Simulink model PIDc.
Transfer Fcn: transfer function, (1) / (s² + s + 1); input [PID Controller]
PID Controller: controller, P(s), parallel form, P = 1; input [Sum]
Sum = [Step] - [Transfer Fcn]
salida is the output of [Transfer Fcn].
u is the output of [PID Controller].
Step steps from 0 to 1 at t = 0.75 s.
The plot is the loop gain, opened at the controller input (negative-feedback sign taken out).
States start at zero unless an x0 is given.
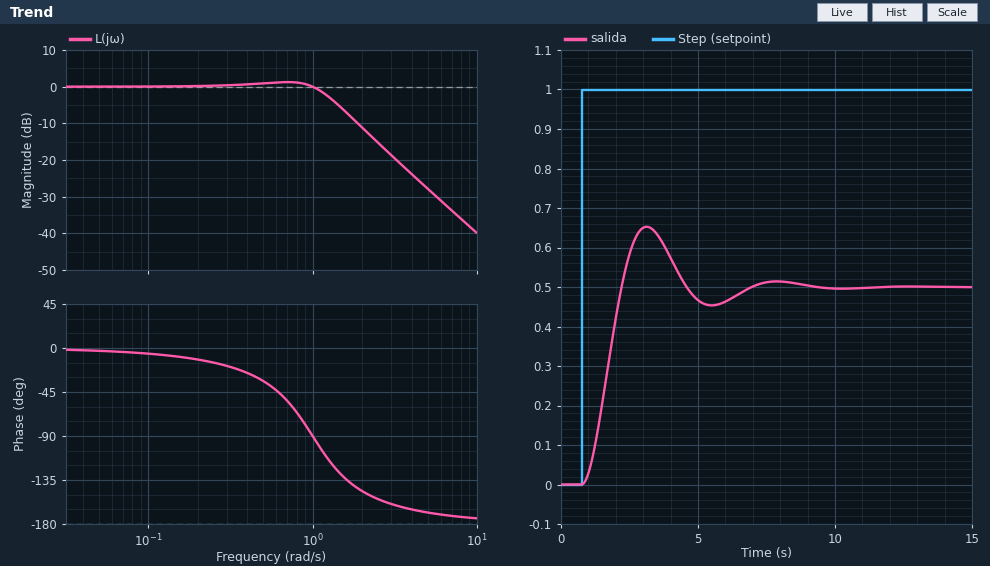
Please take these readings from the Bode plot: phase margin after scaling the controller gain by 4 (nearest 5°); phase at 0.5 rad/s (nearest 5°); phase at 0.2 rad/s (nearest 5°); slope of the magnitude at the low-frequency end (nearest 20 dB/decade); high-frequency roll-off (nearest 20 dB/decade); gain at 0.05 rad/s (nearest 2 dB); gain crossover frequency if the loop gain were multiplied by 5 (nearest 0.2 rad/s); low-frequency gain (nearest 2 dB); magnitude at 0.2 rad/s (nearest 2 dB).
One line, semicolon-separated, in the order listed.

30°; -35°; -10°; 0 dB/decade; -40 dB/decade; 0 dB; 2.4 rad/s; 0 dB; 0 dB
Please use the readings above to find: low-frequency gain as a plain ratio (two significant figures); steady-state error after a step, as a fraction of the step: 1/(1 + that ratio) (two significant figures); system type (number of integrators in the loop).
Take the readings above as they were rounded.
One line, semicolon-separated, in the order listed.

1.0; 0.50; 0
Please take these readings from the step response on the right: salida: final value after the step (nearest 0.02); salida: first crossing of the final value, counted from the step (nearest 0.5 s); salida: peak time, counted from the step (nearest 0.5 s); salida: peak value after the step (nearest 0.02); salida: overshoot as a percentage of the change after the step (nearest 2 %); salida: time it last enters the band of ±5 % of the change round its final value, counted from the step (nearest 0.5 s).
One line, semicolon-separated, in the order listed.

0.50; 1.5 s; 2.5 s; 0.66; 30 %; 5.5 s
